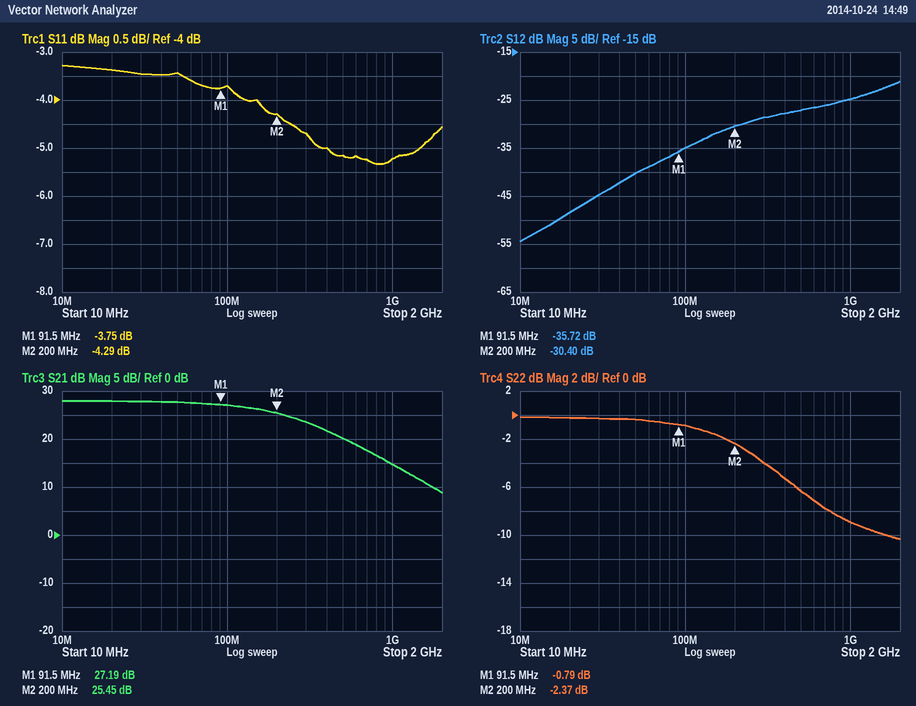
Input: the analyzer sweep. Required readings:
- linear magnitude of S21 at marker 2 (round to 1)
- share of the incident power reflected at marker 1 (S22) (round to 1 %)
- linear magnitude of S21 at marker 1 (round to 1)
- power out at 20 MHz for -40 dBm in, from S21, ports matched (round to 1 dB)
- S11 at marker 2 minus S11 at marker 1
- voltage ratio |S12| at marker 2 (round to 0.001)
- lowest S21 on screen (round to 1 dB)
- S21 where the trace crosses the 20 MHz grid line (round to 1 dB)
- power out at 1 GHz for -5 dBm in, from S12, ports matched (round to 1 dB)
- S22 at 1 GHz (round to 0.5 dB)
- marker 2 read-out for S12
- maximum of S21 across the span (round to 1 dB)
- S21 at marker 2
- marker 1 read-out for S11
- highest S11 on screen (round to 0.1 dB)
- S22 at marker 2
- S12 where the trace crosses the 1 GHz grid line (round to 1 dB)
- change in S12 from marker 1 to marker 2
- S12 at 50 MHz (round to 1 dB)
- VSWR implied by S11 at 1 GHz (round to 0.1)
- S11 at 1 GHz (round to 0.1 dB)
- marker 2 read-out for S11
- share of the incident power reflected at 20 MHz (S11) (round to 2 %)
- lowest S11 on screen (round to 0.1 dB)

19
83 %
23
-12 dBm
-0.54 dB
0.030
9 dB
28 dB
-30 dBm
-9.0 dB
-30.40 dB
28 dB
25.45 dB
-3.75 dB
-3.3 dB
-2.37 dB
-25 dB
5.32 dB
-40 dB
3.4
-5.2 dB
-4.29 dB
46 %
-5.3 dB
